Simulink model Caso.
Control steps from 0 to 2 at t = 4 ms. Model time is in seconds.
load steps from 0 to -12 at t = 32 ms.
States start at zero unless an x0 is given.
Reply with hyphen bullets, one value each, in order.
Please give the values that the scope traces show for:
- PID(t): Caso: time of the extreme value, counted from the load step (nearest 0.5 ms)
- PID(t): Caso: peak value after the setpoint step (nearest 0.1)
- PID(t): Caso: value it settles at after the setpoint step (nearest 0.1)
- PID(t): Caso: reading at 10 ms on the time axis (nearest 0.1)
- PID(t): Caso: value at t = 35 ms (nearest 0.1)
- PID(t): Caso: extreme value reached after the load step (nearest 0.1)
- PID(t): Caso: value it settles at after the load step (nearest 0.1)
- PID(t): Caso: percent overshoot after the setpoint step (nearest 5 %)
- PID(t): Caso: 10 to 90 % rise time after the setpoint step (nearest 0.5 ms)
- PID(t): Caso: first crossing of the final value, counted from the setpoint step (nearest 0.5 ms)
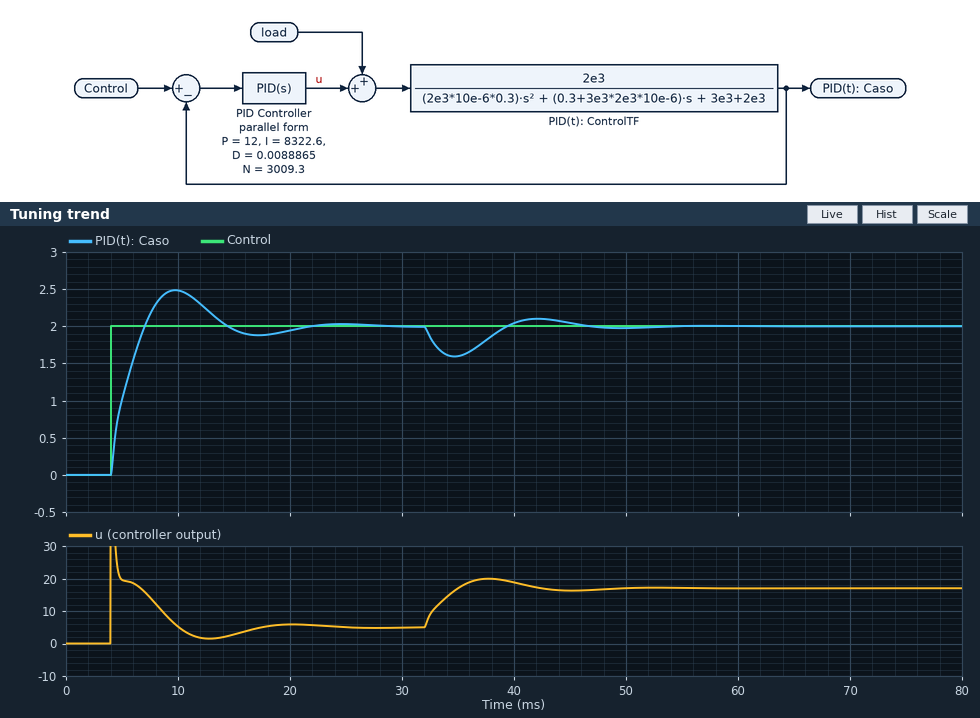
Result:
- 2.5 ms
- 2.5
- 2.0
- 2.5
- 1.6
- 1.6
- 2.0
- 25 %
- 2.5 ms
- 3.0 ms
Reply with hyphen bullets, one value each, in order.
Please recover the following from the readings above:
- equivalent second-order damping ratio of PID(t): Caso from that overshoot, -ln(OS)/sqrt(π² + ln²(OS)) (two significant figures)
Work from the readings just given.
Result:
- 0.40
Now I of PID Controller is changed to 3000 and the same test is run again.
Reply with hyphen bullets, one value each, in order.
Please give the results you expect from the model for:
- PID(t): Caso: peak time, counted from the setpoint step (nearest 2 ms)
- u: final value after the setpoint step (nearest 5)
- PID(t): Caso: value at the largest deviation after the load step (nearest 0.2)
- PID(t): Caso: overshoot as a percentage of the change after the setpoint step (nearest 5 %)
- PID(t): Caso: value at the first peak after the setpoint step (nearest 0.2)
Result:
- 10 ms
- 5
- 1.4
- 10 %
- 2.2
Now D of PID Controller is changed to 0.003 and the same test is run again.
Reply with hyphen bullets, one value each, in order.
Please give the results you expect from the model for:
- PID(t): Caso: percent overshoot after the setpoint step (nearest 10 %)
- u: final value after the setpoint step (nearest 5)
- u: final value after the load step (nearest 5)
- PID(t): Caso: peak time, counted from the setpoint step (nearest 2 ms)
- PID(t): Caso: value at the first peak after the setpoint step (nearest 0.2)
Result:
- 30 %
- 5
- 15
- 6 ms
- 2.6
